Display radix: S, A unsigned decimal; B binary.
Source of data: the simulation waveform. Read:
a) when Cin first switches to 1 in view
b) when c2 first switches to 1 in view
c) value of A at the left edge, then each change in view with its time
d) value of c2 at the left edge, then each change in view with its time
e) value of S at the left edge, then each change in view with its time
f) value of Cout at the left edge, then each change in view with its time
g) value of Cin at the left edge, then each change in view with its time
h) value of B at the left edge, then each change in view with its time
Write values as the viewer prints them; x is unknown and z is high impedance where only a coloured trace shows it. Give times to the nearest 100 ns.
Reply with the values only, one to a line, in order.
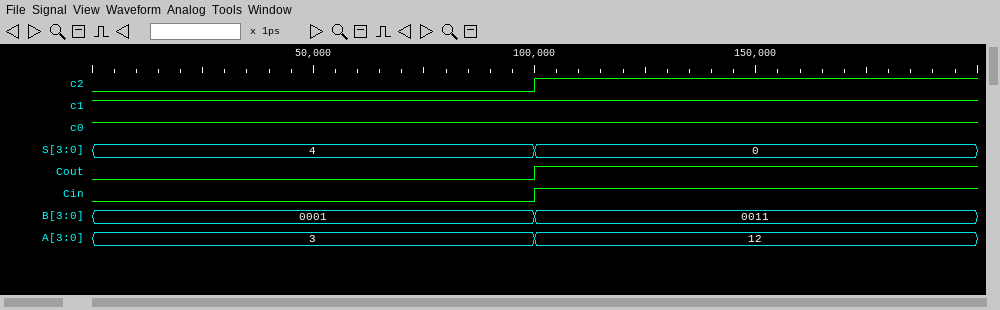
100 ns
100 ns
3, 12 at 100 ns
0, 1 at 100 ns
4, 0 at 100 ns
0, 1 at 100 ns
0, 1 at 100 ns
0001, 0011 at 100 ns
